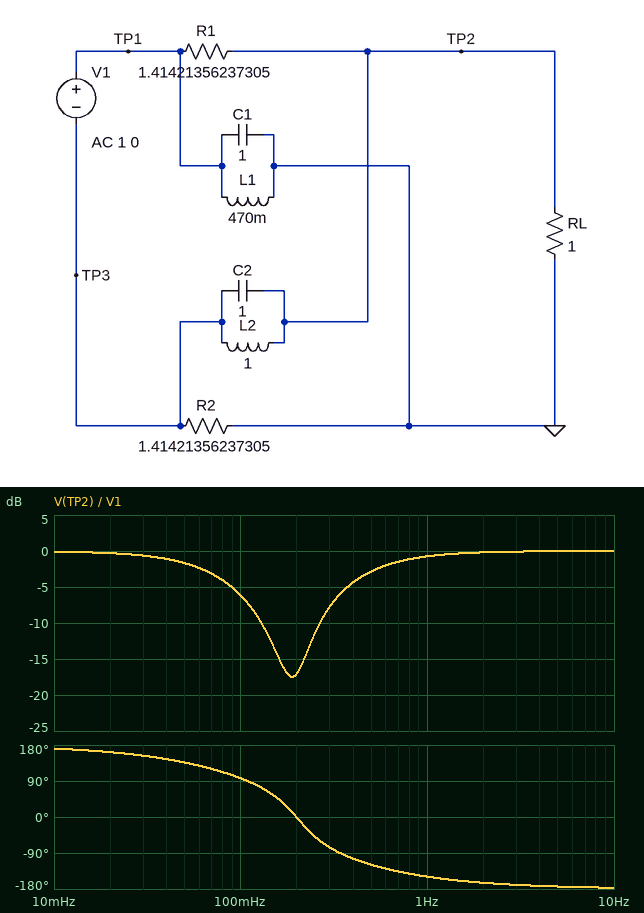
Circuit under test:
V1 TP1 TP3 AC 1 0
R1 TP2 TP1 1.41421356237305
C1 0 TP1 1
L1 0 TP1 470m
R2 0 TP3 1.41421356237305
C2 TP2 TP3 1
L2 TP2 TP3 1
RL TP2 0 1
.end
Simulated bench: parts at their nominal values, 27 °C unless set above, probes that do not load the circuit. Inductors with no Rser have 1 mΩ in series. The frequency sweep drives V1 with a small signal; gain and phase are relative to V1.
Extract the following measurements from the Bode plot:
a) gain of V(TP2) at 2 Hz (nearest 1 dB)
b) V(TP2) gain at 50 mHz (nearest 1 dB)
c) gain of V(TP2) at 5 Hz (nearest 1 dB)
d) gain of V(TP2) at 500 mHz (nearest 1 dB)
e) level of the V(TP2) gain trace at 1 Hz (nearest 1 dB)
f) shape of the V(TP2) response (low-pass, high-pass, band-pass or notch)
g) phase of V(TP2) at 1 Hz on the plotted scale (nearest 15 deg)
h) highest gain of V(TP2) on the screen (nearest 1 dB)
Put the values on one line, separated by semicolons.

0 dB; -2 dB; 0 dB; -3 dB; -1 dB; notch; -150 deg; 0 dB
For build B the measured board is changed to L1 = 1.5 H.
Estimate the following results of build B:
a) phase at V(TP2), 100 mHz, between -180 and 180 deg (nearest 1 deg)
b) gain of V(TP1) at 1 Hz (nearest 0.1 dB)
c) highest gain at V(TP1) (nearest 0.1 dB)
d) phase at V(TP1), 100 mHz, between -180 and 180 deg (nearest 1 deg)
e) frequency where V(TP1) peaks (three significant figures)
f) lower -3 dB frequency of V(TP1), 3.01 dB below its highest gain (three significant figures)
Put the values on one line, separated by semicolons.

58 deg; -11.9 dB; -2.8 dB; 4 deg; 102 mHz; 39.9 mHz
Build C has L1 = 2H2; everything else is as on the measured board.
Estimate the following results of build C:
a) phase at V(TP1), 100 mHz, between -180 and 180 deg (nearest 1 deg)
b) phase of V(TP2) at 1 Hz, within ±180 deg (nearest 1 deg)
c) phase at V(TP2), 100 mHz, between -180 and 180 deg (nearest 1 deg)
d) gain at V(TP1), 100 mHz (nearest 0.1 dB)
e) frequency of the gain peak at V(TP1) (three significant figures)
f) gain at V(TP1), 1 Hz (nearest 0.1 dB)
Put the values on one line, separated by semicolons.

-9 deg; -150 deg; 45 deg; -2.0 dB; 85.4 mHz; -12.0 dB
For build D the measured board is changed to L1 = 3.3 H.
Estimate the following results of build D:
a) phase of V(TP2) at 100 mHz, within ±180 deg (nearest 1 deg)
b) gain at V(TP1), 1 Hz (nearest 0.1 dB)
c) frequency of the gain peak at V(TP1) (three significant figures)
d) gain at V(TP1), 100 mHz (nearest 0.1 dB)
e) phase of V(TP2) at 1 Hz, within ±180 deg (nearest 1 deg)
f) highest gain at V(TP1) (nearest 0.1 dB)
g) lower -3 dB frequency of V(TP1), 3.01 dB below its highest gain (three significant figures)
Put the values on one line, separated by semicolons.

34 deg; -12.0 dB; 72.0 mHz; -1.7 dB; -150 deg; -1.2 dB; 22.8 mHz
